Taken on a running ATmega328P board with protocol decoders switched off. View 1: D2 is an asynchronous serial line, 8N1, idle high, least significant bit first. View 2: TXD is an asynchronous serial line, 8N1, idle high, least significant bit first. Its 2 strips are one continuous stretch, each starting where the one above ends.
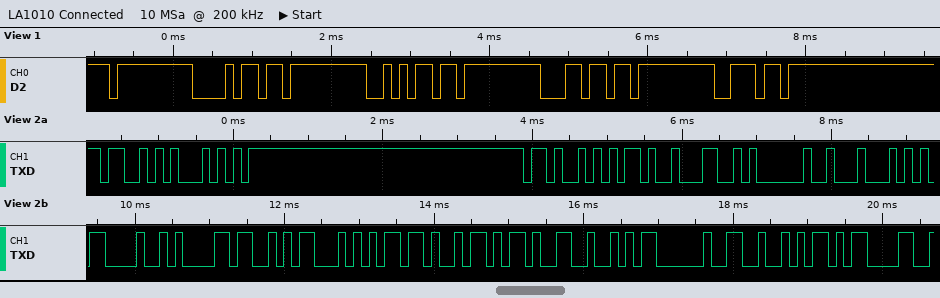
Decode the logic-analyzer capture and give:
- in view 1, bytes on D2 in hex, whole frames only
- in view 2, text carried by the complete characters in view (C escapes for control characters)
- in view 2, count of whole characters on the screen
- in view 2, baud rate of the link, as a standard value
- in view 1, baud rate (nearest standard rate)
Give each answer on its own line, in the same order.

0xFF 0x68 0xFF 0x6A 0xFF 0x6C 0xFF 0x6E
"STK-L D\r\nSTK-R R\r"
17
9600 baud
9600 baud
